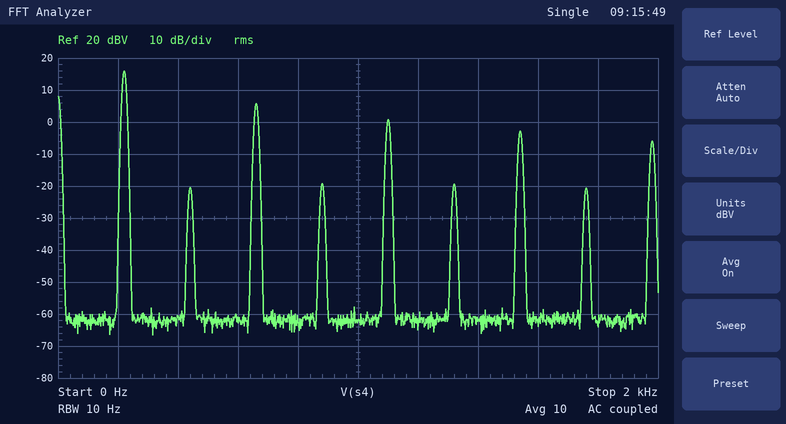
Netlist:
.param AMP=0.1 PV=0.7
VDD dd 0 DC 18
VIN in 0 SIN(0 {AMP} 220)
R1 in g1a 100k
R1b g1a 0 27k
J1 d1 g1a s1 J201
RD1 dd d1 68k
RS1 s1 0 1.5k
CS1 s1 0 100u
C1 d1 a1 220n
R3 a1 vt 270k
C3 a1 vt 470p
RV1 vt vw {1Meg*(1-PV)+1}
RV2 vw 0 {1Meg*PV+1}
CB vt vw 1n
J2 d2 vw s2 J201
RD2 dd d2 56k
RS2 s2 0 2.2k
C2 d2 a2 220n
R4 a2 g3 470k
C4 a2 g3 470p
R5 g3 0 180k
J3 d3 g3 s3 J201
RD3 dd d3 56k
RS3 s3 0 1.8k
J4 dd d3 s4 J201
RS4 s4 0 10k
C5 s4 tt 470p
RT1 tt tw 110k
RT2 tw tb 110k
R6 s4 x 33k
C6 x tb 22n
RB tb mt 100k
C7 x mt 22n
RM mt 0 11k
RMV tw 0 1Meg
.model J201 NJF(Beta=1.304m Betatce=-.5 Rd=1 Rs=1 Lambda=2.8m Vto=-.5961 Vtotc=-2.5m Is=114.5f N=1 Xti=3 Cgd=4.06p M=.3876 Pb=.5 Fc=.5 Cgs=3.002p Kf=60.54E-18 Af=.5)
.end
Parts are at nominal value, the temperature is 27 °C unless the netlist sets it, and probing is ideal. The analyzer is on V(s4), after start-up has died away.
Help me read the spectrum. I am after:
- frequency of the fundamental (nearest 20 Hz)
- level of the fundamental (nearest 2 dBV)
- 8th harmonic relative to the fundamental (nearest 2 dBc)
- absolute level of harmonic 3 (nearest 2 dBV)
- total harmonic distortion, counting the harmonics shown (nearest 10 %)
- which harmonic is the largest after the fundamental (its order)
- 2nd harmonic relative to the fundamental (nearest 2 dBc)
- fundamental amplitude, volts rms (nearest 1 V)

220 Hz
16 dBV
-36 dBc
6 dBV
40 %
3
-36 dBc
6 V
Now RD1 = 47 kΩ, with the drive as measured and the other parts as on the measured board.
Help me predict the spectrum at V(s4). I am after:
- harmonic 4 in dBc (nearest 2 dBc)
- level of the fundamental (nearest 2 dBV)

-40 dBc
16 dBV
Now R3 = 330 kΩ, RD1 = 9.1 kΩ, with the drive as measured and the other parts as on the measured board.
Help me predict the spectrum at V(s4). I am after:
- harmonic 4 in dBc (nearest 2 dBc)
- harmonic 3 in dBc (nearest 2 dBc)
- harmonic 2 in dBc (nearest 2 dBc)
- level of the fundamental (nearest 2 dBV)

-44 dBc
-28 dBc
-20 dBc
14 dBV
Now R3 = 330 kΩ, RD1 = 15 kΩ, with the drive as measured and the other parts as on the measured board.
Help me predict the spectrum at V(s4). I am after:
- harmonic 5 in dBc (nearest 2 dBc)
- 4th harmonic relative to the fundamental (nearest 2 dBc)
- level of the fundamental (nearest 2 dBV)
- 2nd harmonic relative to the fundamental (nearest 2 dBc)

-36 dBc
-28 dBc
16 dBV
-24 dBc
